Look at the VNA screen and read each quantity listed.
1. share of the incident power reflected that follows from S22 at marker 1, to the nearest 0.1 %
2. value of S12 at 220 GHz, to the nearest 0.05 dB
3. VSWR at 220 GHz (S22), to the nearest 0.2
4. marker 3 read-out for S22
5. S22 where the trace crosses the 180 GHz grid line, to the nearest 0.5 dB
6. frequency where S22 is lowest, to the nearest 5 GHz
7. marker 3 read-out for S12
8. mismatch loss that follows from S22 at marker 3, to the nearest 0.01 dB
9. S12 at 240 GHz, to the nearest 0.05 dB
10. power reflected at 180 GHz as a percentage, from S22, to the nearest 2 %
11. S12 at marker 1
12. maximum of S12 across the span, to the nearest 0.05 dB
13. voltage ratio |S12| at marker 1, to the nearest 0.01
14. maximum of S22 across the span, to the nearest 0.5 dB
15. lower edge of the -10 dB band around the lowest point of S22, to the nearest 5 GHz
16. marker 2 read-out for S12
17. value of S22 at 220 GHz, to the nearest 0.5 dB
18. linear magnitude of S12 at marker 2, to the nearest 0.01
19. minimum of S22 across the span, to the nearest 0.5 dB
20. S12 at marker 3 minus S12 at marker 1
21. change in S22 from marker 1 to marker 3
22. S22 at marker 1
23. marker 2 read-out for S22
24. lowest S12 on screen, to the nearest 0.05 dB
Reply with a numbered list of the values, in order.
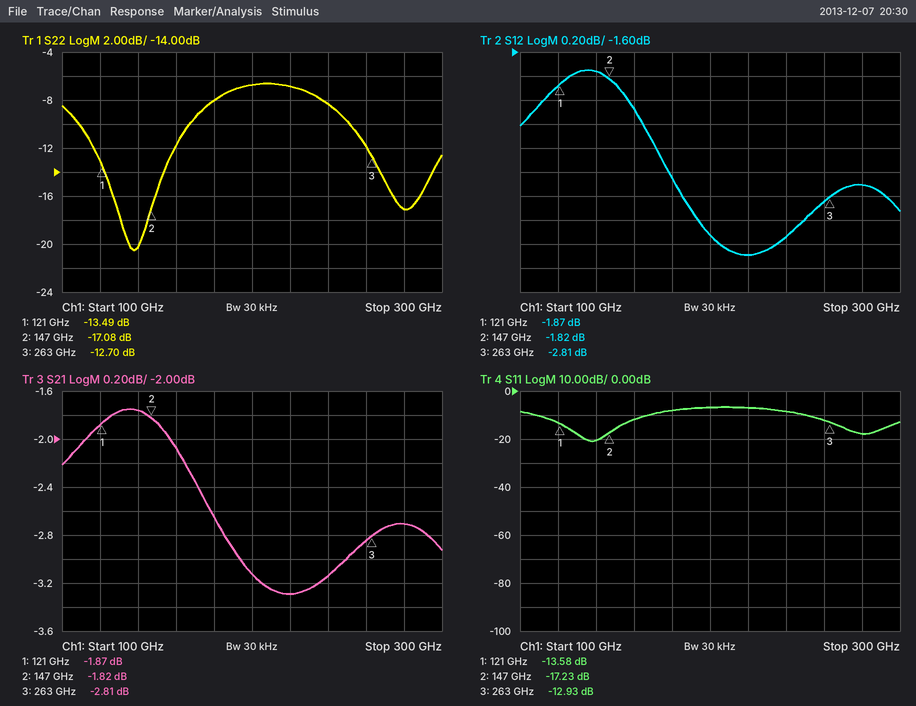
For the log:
1. 4.5 %
2. -3.30 dB
3. 2.6
4. -12.70 dB
5. -8.0 dB
6. 140 GHz
7. -2.81 dB
8. 0.24 dB
9. -3.15 dB
10. 16 %
11. -1.87 dB
12. -1.75 dB
13. 0.81
14. -6.5 dB
15. 110 GHz
16. -1.82 dB
17. -7.0 dB
18. 0.81
19. -20.5 dB
20. -0.94 dB
21. 0.79 dB
22. -13.49 dB
23. -17.08 dB
24. -3.30 dB
